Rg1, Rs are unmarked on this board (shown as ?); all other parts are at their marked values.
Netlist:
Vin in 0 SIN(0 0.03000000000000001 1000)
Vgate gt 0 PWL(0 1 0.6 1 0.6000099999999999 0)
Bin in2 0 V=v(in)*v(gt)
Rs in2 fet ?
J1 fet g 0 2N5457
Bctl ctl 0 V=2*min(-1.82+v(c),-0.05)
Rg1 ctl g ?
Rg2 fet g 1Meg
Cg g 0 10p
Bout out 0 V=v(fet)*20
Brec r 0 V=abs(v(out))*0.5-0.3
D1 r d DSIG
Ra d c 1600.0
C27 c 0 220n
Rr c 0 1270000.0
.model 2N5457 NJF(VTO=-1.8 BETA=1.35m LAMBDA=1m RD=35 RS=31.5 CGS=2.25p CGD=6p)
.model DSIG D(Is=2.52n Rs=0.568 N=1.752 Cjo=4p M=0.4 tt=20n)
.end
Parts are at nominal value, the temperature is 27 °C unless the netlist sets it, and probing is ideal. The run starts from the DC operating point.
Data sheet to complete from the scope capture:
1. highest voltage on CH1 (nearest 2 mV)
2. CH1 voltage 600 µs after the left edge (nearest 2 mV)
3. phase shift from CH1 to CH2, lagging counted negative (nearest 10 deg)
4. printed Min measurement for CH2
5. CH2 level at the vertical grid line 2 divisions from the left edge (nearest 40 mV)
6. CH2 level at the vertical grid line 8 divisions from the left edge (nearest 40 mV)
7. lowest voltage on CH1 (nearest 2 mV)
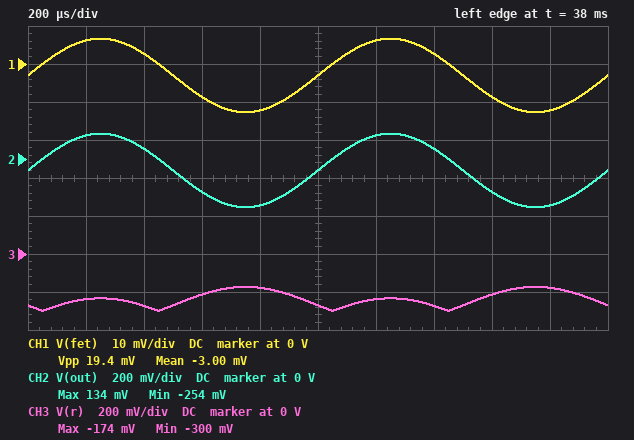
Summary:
6 mV
-8 mV
0 deg
-254 mV
40 mV
-160 mV
-12 mV
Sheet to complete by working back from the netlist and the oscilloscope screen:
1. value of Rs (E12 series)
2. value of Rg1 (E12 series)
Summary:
5.6 kΩ
1.2 MΩ
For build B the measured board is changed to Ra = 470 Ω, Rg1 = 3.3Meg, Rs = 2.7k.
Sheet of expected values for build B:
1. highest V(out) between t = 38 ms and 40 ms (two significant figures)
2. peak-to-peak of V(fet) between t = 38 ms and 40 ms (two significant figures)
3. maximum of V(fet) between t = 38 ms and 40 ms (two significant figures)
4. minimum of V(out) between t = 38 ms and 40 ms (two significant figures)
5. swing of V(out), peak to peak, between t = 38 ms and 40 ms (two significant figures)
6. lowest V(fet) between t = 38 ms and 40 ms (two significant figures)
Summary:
80 mV
8.7 mV
4.0 mV
-93 mV
170 mV
-4.7 mV
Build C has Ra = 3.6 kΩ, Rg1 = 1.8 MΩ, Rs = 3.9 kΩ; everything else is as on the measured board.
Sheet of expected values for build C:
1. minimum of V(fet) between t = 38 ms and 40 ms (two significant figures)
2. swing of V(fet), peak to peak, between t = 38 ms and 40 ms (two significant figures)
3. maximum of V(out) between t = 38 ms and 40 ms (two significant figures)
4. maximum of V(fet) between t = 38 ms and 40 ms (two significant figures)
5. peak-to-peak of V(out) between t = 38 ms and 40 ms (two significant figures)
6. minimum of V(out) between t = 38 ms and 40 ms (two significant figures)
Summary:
-6.0 mV
10 mV
86 mV
4.3 mV
210 mV
-120 mV
